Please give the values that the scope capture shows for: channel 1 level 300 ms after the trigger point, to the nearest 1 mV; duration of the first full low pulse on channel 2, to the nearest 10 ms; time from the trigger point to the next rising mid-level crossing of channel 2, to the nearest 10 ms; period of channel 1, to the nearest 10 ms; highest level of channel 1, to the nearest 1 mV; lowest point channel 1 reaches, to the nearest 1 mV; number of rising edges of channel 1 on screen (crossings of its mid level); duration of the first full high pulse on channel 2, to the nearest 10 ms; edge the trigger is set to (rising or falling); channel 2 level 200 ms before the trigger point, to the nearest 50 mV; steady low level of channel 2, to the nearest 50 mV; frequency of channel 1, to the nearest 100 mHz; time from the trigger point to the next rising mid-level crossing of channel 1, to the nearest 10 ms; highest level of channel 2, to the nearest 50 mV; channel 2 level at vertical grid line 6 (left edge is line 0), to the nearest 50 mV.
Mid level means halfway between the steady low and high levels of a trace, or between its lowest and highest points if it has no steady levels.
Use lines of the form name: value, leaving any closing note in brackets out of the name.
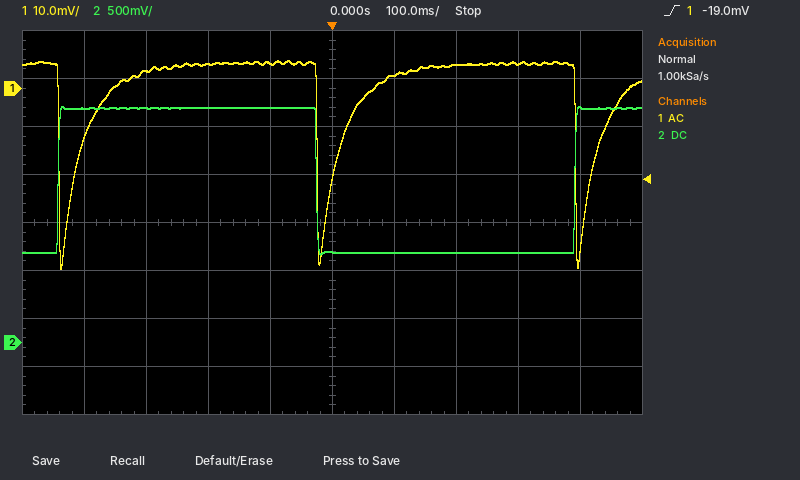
channel 1 level 300 ms after the trigger point, to the nearest 1 mV: 5 mV
duration of the first full low pulse on channel 2, to the nearest 10 ms: 420 ms
time from the trigger point to the next rising mid-level crossing of channel 2, to the nearest 10 ms: 390 ms
period of channel 1, to the nearest 10 ms: 420 ms
highest level of channel 1, to the nearest 1 mV: 6 mV
lowest point channel 1 reaches, to the nearest 1 mV: -38 mV
number of rising edges of channel 1 on screen: 3
duration of the first full high pulse on channel 2, to the nearest 10 ms: 420 ms
edge the trigger is set to: rising
channel 2 level 200 ms before the trigger point, to the nearest 50 mV: 2.45 V
steady low level of channel 2, to the nearest 50 mV: 950 mV
frequency of channel 1, to the nearest 100 mHz: 2.4 Hz
time from the trigger point to the next rising mid-level crossing of channel 1, to the nearest 10 ms: 10 ms
highest level of channel 2, to the nearest 50 mV: 2.45 V
channel 2 level at vertical grid line 6 (left edge is line 0), to the nearest 50 mV: 950 mV
